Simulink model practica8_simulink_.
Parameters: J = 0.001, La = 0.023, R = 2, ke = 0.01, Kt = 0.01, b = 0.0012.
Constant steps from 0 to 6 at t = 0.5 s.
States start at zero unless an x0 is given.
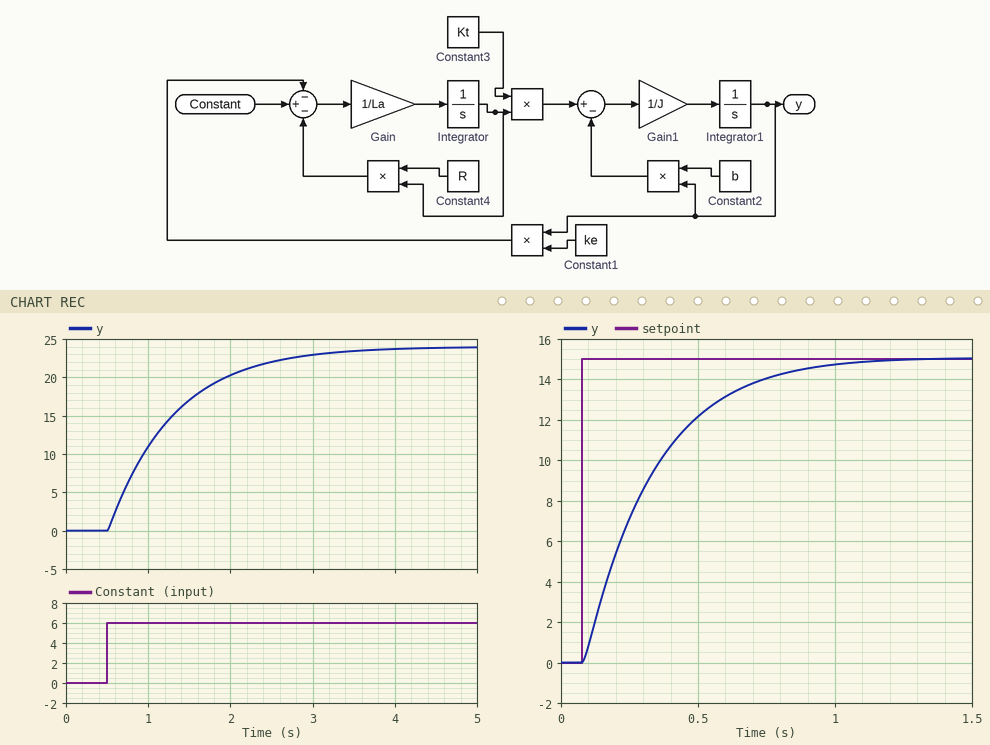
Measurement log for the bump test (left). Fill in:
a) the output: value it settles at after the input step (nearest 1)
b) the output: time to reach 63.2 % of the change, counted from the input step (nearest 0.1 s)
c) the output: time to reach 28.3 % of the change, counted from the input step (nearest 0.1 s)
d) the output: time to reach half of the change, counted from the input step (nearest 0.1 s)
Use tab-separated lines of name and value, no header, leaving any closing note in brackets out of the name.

the output: value it settles at after the input step	24
the output: time to reach 63.2 % of the change, counted from the input step	0.8 s
the output: time to reach 28.3 % of the change, counted from the input step	0.3 s
the output: time to reach half of the change, counted from the input step	0.6 s
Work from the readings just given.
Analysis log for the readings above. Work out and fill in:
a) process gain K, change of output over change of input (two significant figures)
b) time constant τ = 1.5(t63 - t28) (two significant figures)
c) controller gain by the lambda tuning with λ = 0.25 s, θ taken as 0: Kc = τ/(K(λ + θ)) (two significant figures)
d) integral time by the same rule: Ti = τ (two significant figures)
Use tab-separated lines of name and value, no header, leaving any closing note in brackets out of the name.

process gain K, change of output over change of input	4.0
time constant τ = 1.5(t63 - t28)	0.75 s
controller gain by the lambda tuning with λ = 0.25 s, θ taken as 0: Kc = τ/(K(λ + θ))	0.75
integral time by the same rule: Ti = τ	0.75 s
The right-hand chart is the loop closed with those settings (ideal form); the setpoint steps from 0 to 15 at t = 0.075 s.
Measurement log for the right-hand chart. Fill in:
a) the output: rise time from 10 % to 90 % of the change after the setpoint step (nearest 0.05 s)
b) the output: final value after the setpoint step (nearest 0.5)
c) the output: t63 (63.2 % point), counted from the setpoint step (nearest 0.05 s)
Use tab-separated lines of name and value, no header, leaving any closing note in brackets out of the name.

the output: rise time from 10 % to 90 % of the change after the setpoint step	0.55 s
the output: final value after the setpoint step	15.0
the output: t63 (63.2 % point), counted from the setpoint step	0.25 s
